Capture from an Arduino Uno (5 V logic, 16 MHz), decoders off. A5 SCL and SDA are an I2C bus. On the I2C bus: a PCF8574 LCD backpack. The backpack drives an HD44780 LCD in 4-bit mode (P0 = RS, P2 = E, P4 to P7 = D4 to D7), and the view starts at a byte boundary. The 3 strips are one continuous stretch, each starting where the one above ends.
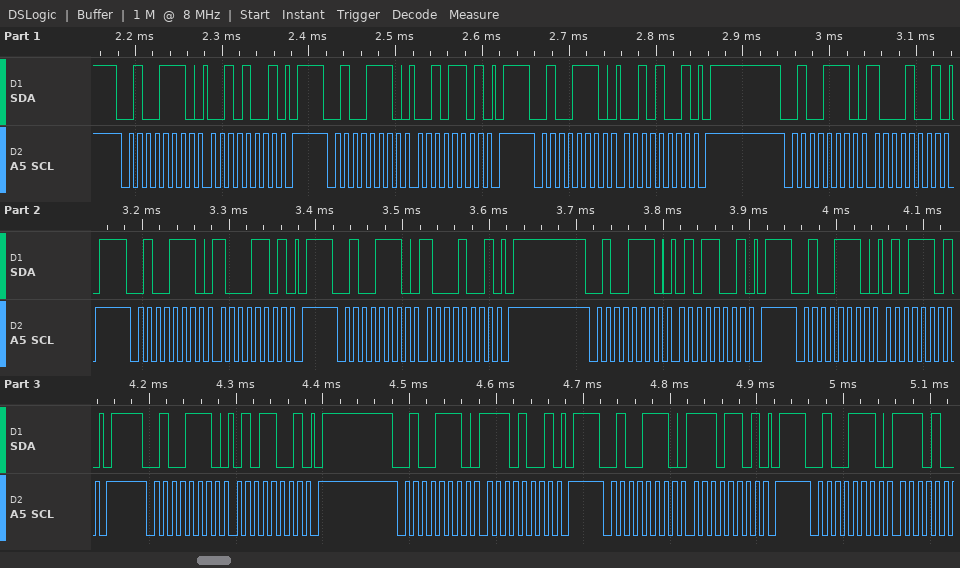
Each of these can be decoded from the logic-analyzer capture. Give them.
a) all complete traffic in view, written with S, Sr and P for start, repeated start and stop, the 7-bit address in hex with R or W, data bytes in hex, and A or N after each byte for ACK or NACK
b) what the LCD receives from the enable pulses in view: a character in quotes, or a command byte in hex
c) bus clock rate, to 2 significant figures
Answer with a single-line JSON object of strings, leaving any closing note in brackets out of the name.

{"all complete traffic in view, written with S, Sr and P for start, repeated start and stop, the 7-bit address in hex with R or W, data bytes in hex, and A or N after each byte for ACK or NACK": "S 27W A 29 A P S 27W A 2D A P S 27W A 29 A P S 27W A 89 A P S 27W A 8D A P S 27W A 89 A P S 27W A 59 A P S 27W A 5D A P S 27W A 59 A P S 27W A E9 A P S 27W A ED A P S 27W A", "what the LCD receives from the enable pulses in view: a character in quotes, or a command byte in hex": "'('", "bus clock rate, to 2 significant figures": "100 kHz"}
